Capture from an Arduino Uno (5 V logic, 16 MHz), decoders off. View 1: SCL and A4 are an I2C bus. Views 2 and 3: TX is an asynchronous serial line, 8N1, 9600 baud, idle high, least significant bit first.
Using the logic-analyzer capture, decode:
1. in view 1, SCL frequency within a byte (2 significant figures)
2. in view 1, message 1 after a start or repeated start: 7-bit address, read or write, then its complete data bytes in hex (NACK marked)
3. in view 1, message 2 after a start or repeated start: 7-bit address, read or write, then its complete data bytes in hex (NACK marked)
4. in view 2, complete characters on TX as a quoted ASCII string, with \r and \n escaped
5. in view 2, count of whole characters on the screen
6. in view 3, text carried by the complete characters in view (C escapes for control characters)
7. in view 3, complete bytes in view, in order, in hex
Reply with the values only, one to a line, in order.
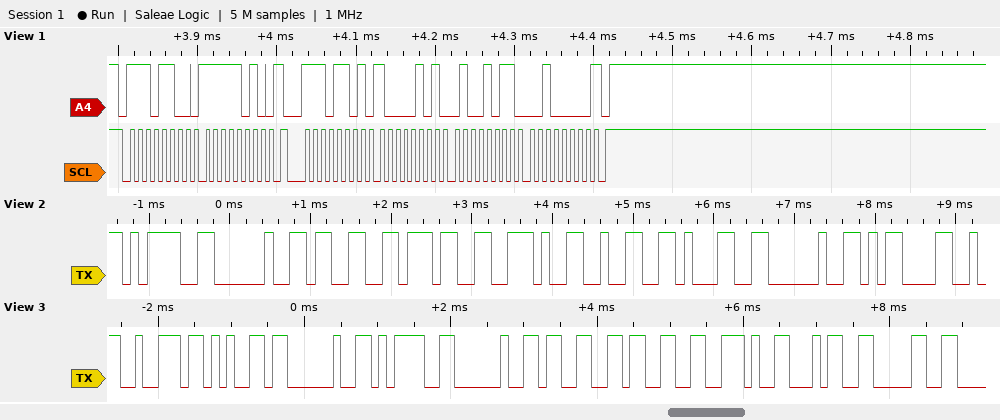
100 kHz
0x76 write: FA
0x76 read: 85 4B 20 NACK
"= 37.21 \r"
9
"re = 33.40"
72 65 20 3D 20 33 33 2E 34 30
